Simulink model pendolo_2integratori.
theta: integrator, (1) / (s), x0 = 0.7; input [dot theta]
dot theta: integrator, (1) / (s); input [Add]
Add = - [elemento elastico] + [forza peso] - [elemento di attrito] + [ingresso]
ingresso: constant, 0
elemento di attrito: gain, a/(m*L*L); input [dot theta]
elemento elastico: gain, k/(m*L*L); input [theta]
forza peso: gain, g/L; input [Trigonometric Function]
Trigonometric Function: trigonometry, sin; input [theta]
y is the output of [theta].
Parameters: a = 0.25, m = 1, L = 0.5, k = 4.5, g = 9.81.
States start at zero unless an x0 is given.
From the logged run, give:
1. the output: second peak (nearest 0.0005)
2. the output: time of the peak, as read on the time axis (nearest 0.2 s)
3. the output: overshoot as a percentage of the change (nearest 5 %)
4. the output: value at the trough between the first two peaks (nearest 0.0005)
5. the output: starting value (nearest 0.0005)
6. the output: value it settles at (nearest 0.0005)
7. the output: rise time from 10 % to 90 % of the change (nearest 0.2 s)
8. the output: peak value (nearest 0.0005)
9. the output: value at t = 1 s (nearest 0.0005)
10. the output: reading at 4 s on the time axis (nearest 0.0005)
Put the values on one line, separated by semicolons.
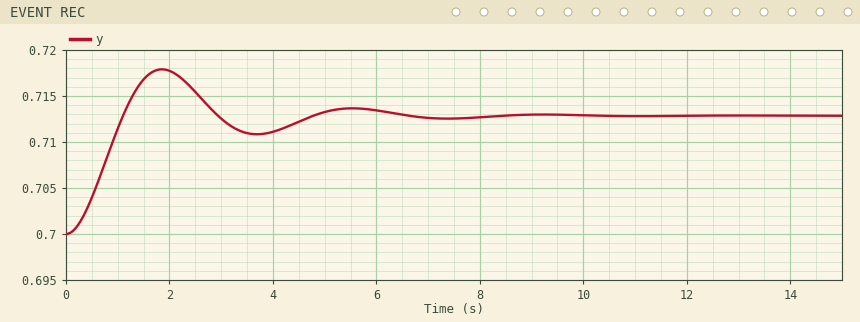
0.7135; 1.8 s; 40 %; 0.7110; 0.7000; 0.7130; 0.8 s; 0.7180; 0.7115; 0.7110
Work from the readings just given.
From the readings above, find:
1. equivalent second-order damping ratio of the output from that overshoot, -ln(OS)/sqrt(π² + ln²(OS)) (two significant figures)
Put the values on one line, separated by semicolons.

0.28
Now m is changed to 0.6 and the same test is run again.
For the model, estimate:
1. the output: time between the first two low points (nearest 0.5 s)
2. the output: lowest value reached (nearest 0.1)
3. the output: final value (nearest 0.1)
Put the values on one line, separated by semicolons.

2.0 s; -0.3; 0.0
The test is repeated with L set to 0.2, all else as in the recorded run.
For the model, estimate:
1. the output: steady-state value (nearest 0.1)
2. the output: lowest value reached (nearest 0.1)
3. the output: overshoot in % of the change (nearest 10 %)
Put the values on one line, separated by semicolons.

0.0; -0.2; 30 %
